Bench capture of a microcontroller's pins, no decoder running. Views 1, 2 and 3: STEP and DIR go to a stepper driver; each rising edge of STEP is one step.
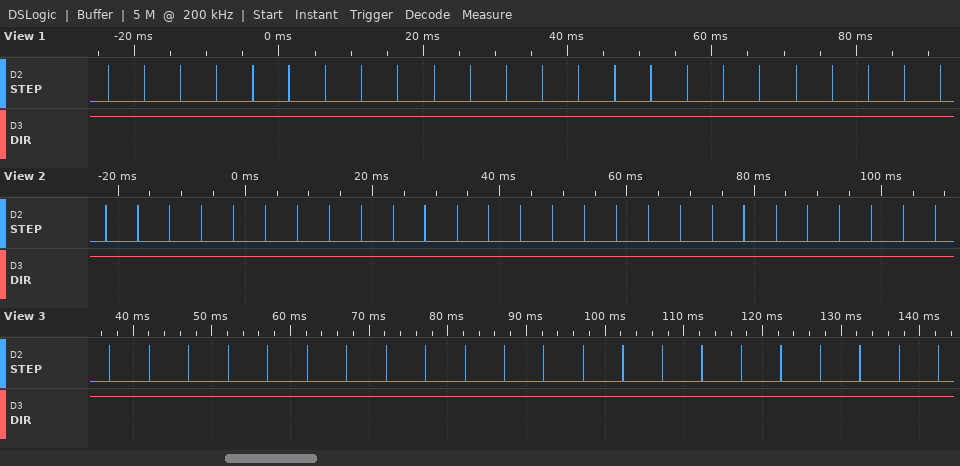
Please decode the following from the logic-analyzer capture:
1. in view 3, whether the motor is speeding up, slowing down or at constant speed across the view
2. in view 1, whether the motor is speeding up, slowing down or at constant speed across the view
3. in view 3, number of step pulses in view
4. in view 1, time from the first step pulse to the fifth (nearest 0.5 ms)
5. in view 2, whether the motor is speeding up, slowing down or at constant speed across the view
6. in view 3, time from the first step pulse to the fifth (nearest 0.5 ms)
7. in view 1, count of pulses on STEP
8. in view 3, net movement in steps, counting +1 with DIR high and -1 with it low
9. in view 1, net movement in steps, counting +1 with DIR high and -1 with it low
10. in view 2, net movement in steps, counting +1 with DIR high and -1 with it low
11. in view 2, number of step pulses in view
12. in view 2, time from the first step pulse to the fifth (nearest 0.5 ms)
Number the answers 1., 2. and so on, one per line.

1. constant speed
2. constant speed
3. 22
4. 20.0 ms
5. constant speed
6. 20.0 ms
7. 24
8. +22
9. +24
10. +27
11. 27
12. 20.0 ms
